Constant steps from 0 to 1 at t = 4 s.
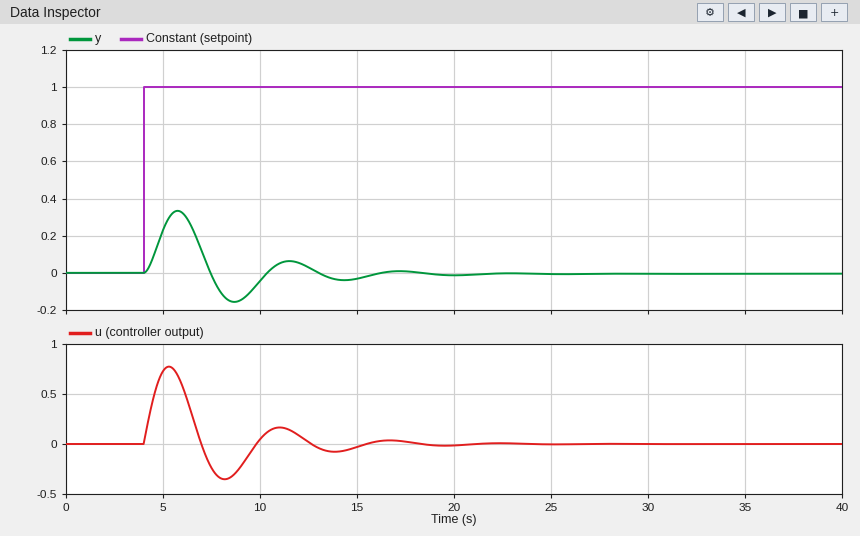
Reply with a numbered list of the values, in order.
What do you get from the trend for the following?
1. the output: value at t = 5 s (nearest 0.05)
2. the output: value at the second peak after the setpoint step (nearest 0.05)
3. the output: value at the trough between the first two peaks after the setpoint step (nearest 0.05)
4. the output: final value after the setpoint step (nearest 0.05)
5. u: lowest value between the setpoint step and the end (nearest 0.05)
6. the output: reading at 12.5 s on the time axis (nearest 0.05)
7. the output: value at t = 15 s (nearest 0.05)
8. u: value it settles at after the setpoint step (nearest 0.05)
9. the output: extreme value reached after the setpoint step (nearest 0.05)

1. 0.25
2. 0.05
3. -0.15
4. 0.00
5. -0.35
6. 0.05
7. -0.05
8. 0.00
9. 0.35
